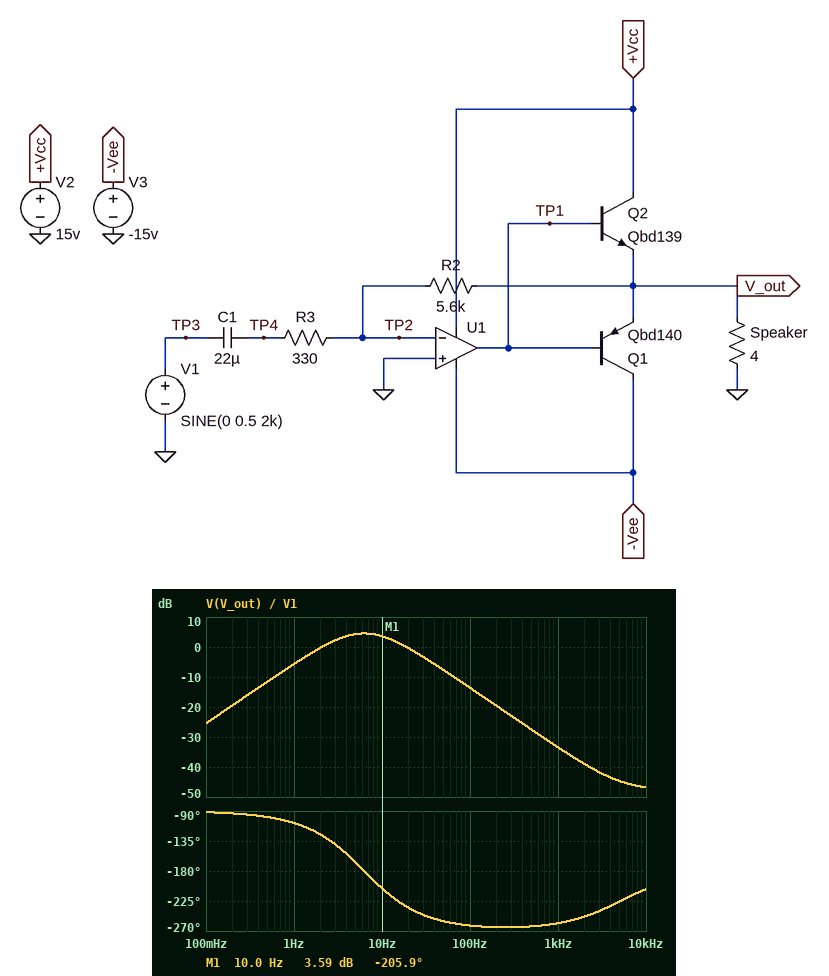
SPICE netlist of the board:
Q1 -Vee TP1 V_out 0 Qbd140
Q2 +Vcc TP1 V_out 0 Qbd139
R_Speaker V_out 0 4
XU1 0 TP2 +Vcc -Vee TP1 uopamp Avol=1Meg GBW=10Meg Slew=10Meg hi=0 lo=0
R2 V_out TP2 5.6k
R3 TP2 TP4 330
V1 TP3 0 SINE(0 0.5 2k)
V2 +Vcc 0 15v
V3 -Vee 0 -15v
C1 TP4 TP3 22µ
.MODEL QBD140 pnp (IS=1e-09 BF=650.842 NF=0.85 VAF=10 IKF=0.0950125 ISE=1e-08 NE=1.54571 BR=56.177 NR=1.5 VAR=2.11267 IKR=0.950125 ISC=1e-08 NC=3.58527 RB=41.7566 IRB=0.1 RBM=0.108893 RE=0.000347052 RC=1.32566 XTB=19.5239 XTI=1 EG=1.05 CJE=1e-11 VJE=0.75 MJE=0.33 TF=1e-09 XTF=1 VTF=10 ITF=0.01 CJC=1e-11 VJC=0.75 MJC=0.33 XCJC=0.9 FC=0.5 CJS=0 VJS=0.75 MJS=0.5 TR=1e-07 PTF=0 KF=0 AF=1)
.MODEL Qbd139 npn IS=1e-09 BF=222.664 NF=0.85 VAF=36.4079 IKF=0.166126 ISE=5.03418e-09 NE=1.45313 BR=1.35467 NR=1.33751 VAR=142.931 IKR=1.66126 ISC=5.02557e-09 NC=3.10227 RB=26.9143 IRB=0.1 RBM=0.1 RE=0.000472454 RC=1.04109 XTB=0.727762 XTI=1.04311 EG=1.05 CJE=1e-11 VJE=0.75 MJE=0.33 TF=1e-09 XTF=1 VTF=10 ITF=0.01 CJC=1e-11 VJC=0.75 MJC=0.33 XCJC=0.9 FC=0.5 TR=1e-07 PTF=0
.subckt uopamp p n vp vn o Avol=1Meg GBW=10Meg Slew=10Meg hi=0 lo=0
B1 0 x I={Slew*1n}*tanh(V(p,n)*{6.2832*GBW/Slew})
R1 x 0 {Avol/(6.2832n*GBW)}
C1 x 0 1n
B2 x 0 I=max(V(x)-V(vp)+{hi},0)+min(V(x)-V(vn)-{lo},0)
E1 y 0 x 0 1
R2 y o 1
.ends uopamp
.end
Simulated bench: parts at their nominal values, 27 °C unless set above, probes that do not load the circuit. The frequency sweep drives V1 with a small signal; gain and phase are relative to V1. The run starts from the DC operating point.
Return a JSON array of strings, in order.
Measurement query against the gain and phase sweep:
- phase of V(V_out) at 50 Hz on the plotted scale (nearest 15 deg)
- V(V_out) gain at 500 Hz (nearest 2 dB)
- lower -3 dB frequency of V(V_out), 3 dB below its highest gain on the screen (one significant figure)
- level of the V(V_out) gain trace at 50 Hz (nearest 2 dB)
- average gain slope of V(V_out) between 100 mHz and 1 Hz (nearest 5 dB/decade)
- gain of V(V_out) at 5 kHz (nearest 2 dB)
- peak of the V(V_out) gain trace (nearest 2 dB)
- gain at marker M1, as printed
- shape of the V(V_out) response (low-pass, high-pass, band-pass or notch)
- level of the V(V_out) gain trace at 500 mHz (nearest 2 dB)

["-255 deg", "-28 dB", "3 Hz", "-8 dB", "20 dB/decade", "-44 dB", "4 dB", "3.59 dB", "band-pass", "-12 dB"]
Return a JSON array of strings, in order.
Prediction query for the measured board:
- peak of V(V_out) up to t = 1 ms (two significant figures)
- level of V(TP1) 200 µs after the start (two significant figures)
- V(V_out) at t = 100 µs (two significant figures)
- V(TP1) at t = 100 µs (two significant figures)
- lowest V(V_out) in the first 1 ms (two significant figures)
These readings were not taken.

["8.6 V", "-5.8 V", "-8.0 V", "-9.9 V", "-8.4 V"]
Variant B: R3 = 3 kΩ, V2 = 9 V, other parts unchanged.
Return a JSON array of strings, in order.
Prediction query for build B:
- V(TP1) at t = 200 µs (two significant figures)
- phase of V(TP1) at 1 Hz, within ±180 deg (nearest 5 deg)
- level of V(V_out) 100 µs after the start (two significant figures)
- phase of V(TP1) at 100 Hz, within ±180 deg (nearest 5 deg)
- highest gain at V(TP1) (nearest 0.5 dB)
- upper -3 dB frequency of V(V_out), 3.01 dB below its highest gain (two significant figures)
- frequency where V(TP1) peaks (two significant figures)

["-970 mV", "-125 deg", "-890 mV", "100 deg", "111.0 dB", "20 Hz", "5.2 Hz"]
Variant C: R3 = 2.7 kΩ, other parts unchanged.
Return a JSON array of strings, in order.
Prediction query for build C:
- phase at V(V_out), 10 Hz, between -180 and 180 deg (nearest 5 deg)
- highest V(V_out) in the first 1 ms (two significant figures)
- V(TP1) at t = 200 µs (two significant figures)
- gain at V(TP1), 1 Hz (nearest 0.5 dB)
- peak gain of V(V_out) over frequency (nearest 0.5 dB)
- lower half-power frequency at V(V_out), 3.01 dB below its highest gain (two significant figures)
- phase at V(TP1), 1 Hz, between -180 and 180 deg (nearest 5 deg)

["160 deg", "1.0 V", "-1.0 V", "106.5 dB", "-1.5 dB", "1.4 Hz", "-125 deg"]
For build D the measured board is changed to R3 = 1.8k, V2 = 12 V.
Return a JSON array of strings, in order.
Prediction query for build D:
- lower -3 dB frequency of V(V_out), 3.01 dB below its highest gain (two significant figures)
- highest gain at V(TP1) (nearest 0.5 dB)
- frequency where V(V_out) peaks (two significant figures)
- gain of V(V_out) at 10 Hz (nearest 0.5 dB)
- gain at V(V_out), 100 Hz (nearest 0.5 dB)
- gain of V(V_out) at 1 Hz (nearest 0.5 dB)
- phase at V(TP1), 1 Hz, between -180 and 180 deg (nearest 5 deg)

["1.7 Hz", "113.5 dB", "5.6 Hz", "-0.5 dB", "-15.5 dB", "-6.5 dB", "-120 deg"]
